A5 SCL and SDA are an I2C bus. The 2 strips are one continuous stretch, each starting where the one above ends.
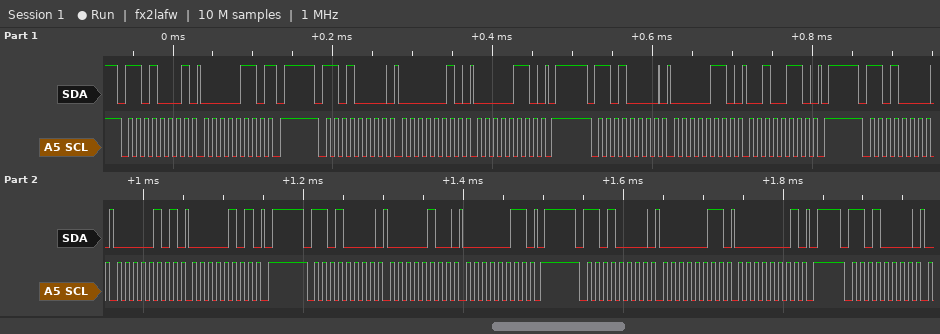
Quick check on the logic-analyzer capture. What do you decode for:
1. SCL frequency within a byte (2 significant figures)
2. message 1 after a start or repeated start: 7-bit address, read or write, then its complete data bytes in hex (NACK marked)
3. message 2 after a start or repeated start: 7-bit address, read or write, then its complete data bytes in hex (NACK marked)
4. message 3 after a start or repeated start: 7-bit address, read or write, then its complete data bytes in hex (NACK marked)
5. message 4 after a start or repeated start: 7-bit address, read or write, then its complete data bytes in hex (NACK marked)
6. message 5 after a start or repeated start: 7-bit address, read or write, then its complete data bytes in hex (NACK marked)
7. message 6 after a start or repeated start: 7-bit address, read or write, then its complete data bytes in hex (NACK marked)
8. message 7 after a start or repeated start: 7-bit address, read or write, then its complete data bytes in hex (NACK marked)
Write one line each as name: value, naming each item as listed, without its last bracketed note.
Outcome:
SCL frequency within a byte: 100 kHz
message 1 after a start or repeated start: 7-bit address, read or write, then its complete data bytes in hex: 0x68 read: 06 NACK
message 2 after a start or repeated start: 7-bit address, read or write, then its complete data bytes in hex: 0x68 write: 02 06
message 3 after a start or repeated start: 7-bit address, read or write, then its complete data bytes in hex: 0x68 write: 06 26
message 4 after a start or repeated start: 7-bit address, read or write, then its complete data bytes in hex: 0x68 write: 05 05
message 5 after a start or repeated start: 7-bit address, read or write, then its complete data bytes in hex: 0x68 write: 04 03
message 6 after a start or repeated start: 7-bit address, read or write, then its complete data bytes in hex: 0x68 write: 03 01
message 7 after a start or repeated start: 7-bit address, read or write, then its complete data bytes in hex: 0x68 write
